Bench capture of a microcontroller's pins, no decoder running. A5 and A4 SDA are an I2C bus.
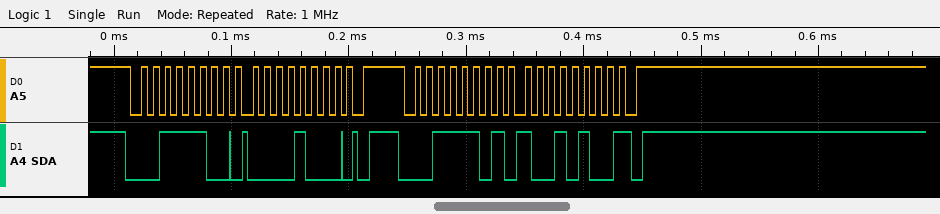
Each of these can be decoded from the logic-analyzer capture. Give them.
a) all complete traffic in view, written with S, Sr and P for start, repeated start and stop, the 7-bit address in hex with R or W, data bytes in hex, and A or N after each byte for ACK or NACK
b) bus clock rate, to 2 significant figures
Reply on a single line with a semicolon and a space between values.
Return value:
S 1EW A 08 A P S 1ER A 94 N P; 100 kHz
